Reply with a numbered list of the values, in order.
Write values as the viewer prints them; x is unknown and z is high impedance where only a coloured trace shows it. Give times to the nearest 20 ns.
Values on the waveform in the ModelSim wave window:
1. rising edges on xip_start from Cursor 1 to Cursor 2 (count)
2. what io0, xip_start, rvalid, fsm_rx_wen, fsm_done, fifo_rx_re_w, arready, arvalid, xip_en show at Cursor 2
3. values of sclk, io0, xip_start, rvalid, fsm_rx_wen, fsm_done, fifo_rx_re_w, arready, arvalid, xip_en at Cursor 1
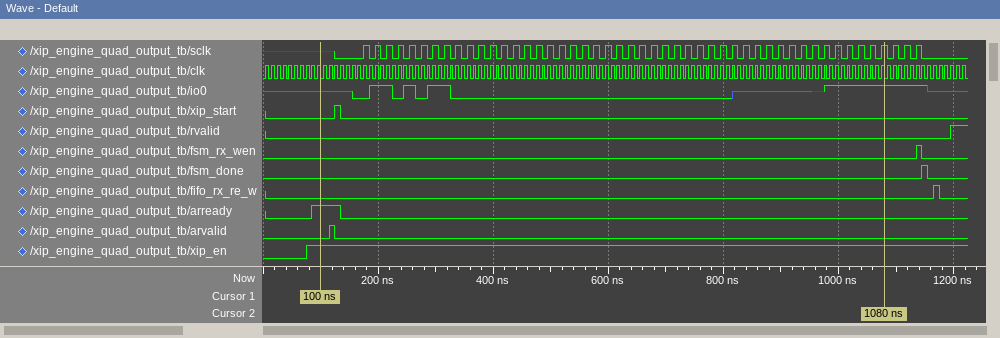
1. 1
2. io0=1, xip_start=0, rvalid=0, fsm_rx_wen=0, fsm_done=0, fifo_rx_re_w=0, arready=0, arvalid=0, xip_en=1
3. sclk=x, io0=z, xip_start=0, rvalid=0, fsm_rx_wen=0, fsm_done=0, fifo_rx_re_w=0, arready=1, arvalid=0, xip_en=1
